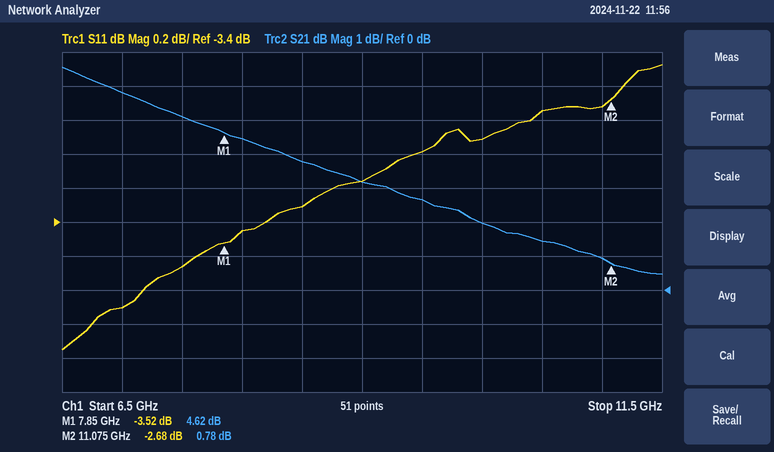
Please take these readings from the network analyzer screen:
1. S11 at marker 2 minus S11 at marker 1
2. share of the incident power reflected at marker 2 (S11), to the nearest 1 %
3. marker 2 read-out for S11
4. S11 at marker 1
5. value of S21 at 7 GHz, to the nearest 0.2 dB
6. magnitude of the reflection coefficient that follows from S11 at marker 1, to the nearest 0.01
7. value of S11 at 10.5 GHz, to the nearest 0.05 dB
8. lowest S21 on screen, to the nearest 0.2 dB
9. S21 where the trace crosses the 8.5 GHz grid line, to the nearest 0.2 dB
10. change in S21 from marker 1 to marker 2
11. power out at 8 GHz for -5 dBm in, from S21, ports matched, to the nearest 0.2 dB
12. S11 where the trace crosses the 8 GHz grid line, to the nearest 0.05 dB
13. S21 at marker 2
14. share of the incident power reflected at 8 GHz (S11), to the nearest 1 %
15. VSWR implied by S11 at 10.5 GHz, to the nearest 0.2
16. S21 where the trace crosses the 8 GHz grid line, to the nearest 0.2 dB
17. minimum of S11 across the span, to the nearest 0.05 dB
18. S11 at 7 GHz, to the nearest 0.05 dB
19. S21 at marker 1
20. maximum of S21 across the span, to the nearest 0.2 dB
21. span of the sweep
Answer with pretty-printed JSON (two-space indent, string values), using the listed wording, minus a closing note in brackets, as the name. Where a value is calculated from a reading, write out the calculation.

{
  "S11 at marker 2 minus S11 at marker 1": "-2.68 − (-3.52) = 0.84 dB",
  "share of the incident power reflected at marker 2 (S11), to the nearest 1 %": "10^(-2.68/10) ≈ 54 %",
  "marker 2 read-out for S11": "-2.68 dB",
  "S11 at marker 1": "-3.52 dB",
  "value of S21 at 7 GHz, to the nearest 0.2 dB": "5.8 dB",
  "magnitude of the reflection coefficient that follows from S11 at marker 1, to the nearest 0.01": "10^(-3.52/20) ≈ 0.67",
  "value of S11 at 10.5 GHz, to the nearest 0.05 dB": "-2.75 dB",
  "lowest S21 on screen, to the nearest 0.2 dB": "0.4 dB",
  "S21 where the trace crosses the 8.5 GHz grid line, to the nearest 0.2 dB": "3.8 dB",
  "change in S21 from marker 1 to marker 2": "0.78 − (4.62) = -3.84 dB",
  "power out at 8 GHz for -5 dBm in, from S21, ports matched, to the nearest 0.2 dB": "-5 dBm + (4.4 dB) = -0.6 dBm",
  "S11 where the trace crosses the 8 GHz grid line, to the nearest 0.05 dB": "-3.45 dB",
  "S21 at marker 2": "0.78 dB",
  "share of the incident power reflected at 8 GHz (S11), to the nearest 1 %": "10^(-3.45/10) ≈ 45 %",
  "VSWR implied by S11 at 10.5 GHz, to the nearest 0.2": "|Γ| = 10^(-2.75/20) = 0.7286; VSWR = (1 + 0.7286)/(1 − 0.7286) ≈ 6.4",
  "S21 where the trace crosses the 8 GHz grid line, to the nearest 0.2 dB": "4.4 dB",
  "minimum of S11 across the span, to the nearest 0.05 dB": "-4.15 dB",
  "S11 at 7 GHz, to the nearest 0.05 dB": "-3.90 dB",
  "S21 at marker 1": "4.62 dB",
  "maximum of S21 across the span, to the nearest 0.2 dB": "6.6 dB",
  "span of the sweep": "5 GHz"
}
